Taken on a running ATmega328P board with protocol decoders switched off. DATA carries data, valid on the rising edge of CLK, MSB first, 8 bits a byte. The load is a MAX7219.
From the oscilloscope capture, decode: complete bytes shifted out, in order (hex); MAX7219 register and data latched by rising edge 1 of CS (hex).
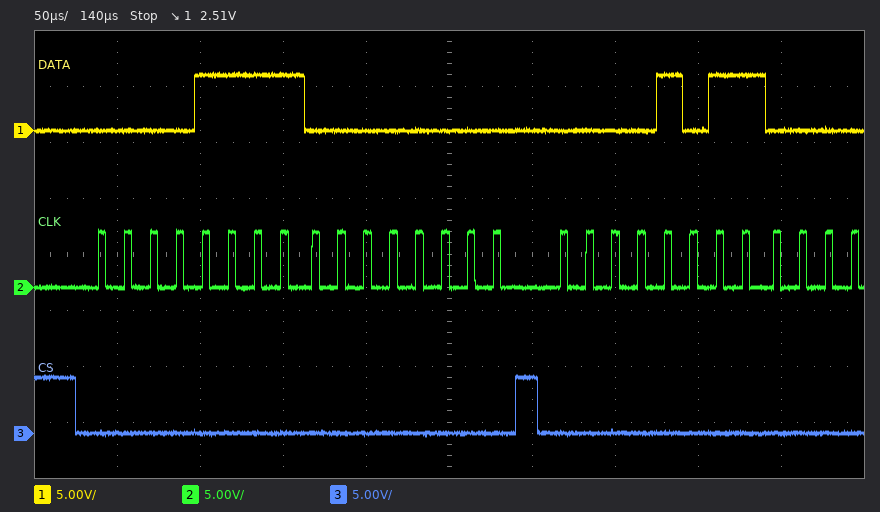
0F 00 0B
register 0xF, data 0x00
